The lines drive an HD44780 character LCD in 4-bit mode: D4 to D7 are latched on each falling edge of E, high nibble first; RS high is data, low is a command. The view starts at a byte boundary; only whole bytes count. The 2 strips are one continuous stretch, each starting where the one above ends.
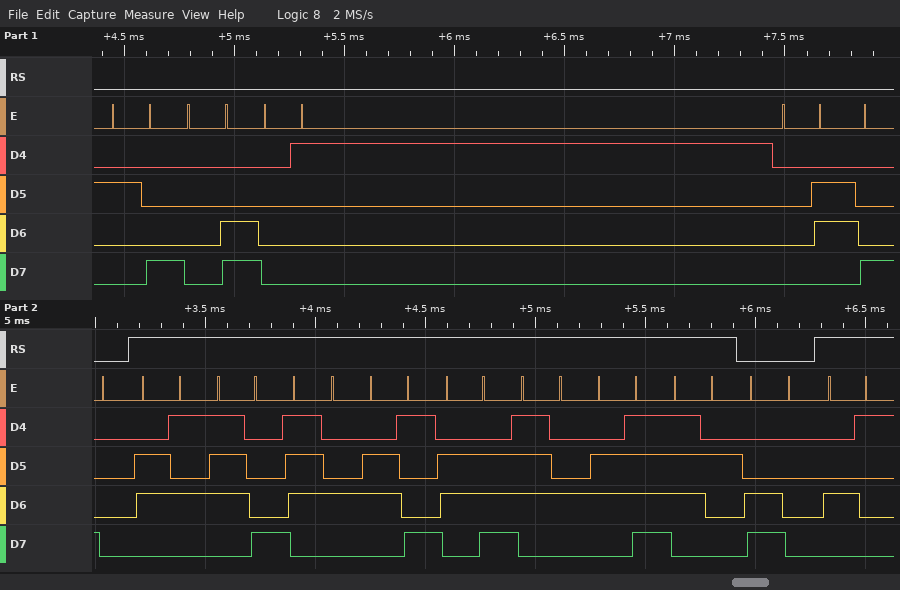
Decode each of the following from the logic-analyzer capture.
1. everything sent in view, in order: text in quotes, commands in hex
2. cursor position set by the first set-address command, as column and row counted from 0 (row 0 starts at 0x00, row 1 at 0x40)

0x28 0x0C 0x01 0x06 0x80 "extintor" 0xC0 "A"
column 0, row 0
